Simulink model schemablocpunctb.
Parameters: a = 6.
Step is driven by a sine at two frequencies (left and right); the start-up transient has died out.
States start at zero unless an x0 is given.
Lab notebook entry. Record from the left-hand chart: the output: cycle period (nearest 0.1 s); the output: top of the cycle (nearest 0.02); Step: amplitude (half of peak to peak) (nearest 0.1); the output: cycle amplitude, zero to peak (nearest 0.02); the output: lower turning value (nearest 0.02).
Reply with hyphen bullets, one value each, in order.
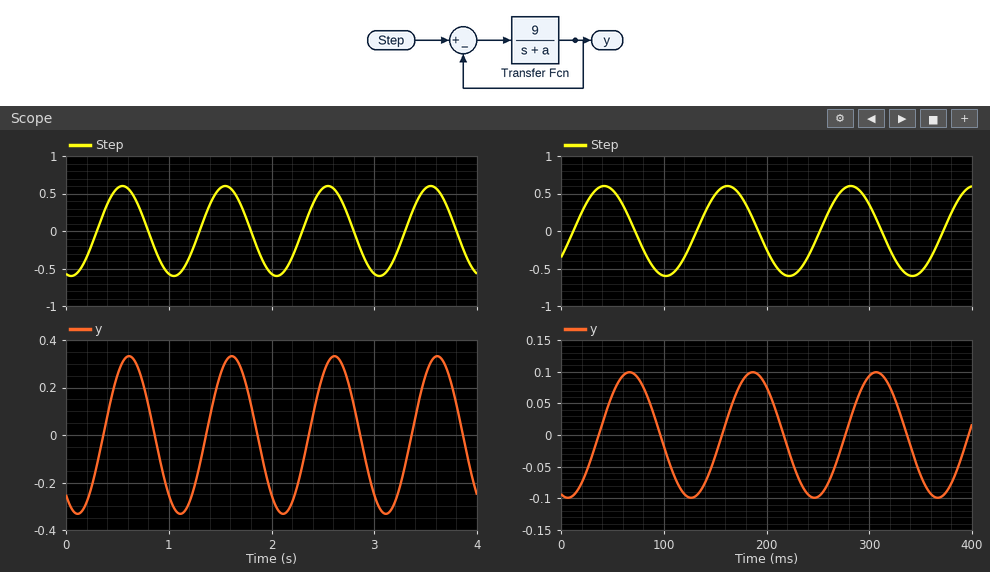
- 1.0 s
- 0.34
- 0.6
- 0.34
- -0.34
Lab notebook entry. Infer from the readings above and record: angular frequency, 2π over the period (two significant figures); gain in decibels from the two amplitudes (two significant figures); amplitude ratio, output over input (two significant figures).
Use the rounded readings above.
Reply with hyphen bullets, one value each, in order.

- 6.3 rad/s
- -4.9 dB
- 0.57
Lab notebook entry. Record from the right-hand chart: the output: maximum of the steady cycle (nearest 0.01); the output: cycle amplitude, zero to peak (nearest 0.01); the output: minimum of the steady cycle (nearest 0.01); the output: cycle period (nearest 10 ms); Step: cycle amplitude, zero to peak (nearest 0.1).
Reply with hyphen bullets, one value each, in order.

- 0.10
- 0.10
- -0.10
- 120 ms
- 0.6
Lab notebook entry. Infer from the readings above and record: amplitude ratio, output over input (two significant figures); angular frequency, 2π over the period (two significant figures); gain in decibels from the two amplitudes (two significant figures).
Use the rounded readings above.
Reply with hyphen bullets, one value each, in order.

- 0.17
- 0.052 rad/ms
- -16 dB
